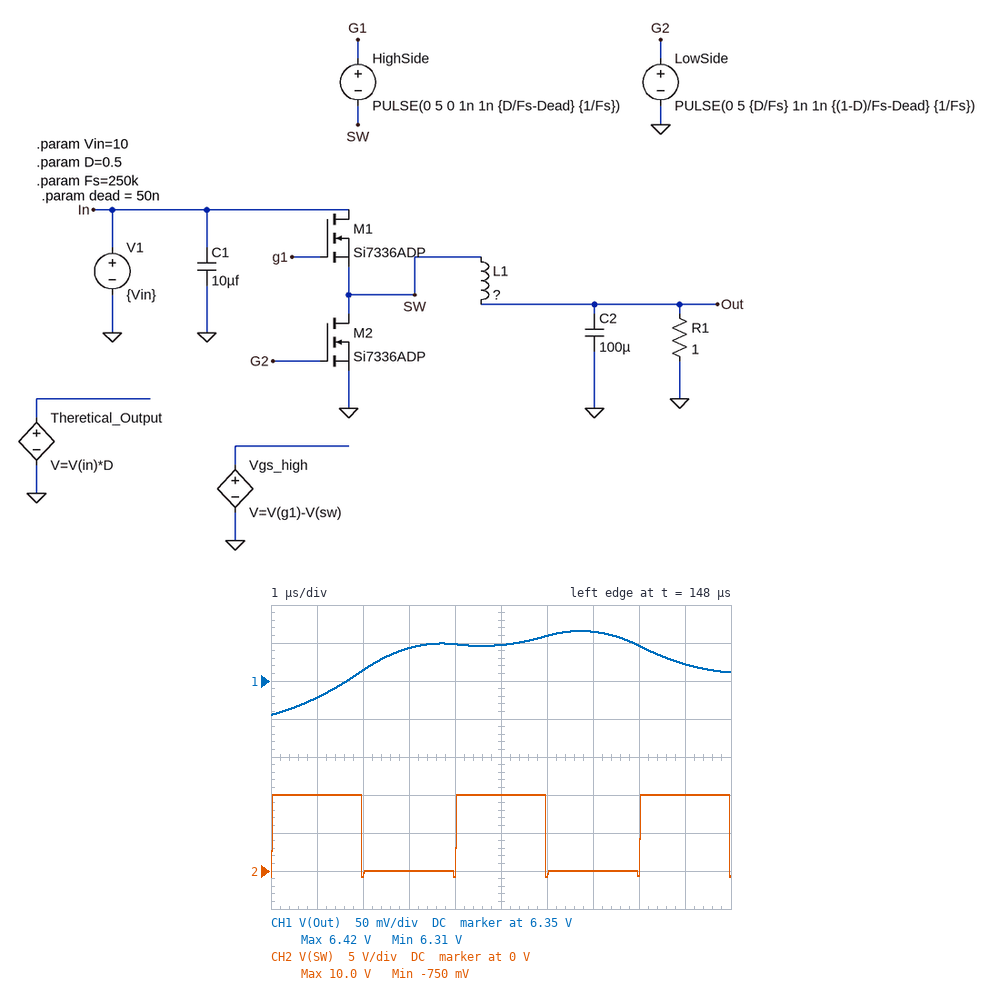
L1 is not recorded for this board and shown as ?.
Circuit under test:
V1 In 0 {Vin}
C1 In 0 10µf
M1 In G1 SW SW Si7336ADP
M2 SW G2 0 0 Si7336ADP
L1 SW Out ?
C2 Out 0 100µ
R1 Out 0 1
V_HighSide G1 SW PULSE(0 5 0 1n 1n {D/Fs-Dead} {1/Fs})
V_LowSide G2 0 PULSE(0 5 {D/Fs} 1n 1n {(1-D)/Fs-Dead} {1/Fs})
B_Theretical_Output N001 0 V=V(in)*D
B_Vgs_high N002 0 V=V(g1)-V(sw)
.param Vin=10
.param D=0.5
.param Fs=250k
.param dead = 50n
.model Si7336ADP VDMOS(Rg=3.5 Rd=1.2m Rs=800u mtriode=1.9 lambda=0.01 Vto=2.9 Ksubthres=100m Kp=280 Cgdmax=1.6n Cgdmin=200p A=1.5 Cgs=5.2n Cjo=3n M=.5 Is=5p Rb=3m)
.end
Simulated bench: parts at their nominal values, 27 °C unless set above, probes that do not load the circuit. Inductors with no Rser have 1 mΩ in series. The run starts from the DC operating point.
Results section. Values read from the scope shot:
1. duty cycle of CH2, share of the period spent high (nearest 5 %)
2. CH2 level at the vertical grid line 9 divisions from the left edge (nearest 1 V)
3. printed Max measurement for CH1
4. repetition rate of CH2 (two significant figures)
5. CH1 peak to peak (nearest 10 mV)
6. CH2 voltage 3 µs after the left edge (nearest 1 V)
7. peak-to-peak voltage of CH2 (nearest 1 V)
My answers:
50 %
10 V
6.42 V
250 kHz
110 mV
0 V
11 V
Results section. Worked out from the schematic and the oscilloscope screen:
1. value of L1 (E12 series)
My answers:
2.7 µH
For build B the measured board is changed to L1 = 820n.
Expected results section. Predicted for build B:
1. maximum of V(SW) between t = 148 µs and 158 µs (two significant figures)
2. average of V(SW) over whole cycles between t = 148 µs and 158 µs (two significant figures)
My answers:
11 V
5.0 V
